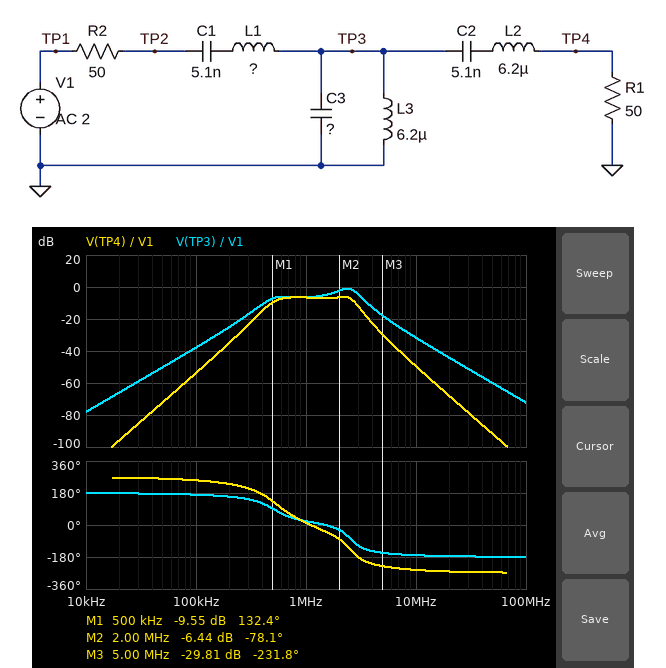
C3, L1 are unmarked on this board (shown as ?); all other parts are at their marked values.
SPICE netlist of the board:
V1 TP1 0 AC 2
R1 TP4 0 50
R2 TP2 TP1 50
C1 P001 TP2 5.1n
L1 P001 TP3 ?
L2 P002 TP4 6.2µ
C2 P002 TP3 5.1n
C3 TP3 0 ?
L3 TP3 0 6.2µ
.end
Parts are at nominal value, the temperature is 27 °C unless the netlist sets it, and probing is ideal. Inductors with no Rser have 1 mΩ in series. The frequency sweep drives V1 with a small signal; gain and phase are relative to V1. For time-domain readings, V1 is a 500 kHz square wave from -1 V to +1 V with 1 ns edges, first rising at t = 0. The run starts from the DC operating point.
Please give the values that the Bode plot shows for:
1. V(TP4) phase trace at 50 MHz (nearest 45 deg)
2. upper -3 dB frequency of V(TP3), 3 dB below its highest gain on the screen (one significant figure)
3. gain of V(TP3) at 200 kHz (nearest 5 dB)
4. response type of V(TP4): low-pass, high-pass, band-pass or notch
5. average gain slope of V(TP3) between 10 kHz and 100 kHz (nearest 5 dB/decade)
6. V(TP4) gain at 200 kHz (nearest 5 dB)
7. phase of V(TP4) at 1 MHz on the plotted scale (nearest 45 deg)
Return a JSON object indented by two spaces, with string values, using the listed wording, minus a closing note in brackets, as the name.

{
  "V(TP4) phase trace at 50 MHz": "-270 deg",
  "upper -3 dB frequency of V(TP3), 3 dB below its highest gain on the screen": "3 MHz",
  "gain of V(TP3) at 200 kHz": "-25 dB",
  "response type of V(TP4): low-pass, high-pass, band-pass or notch": "band-pass",
  "average gain slope of V(TP3) between 10 kHz and 100 kHz": "40 dB/decade",
  "V(TP4) gain at 200 kHz": "-35 dB",
  "phase of V(TP4) at 1 MHz on the plotted scale": "0 deg"
}
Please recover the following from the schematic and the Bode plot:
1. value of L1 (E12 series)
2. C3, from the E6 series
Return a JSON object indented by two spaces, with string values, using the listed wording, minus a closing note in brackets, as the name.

{
  "value of L1": "4.7 µH",
  "C3, from the E6 series": "2.2 nF"
}
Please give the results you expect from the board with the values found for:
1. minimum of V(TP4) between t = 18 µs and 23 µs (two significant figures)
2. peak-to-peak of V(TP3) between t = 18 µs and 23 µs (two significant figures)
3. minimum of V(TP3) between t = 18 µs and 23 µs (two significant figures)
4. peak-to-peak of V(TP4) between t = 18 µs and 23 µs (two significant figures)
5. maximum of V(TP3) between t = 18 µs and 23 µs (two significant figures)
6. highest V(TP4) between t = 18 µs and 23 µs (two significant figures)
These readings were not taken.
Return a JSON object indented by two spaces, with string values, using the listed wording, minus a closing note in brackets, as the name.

{
  "minimum of V(TP4) between t = 18 µs and 23 µs": "-510 mV",
  "peak-to-peak of V(TP3) between t = 18 µs and 23 µs": "2.0 V",
  "minimum of V(TP3) between t = 18 µs and 23 µs": "-1.0 V",
  "peak-to-peak of V(TP4) between t = 18 µs and 23 µs": "1.0 V",
  "maximum of V(TP3) between t = 18 µs and 23 µs": "1.0 V",
  "highest V(TP4) between t = 18 µs and 23 µs": "510 mV"
}
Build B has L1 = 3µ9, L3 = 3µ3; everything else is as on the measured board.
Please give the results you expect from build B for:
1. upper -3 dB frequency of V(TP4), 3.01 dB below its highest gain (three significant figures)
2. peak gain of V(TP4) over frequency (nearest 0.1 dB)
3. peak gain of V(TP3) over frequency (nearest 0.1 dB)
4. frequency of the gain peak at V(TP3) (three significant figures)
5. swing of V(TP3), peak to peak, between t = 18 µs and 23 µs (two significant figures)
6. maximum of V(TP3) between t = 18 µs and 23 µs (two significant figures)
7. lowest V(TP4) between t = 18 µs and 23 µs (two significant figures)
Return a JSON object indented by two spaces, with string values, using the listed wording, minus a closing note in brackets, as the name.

{
  "upper -3 dB frequency of V(TP4), 3.01 dB below its highest gain": "3.11 MHz",
  "peak gain of V(TP4) over frequency": "-6.6 dB",
  "peak gain of V(TP3) over frequency": "0 dB",
  "frequency of the gain peak at V(TP3)": "2.75 MHz",
  "swing of V(TP3), peak to peak, between t = 18 µs and 23 µs": "1.4 V",
  "maximum of V(TP3) between t = 18 µs and 23 µs": "690 mV",
  "lowest V(TP4) between t = 18 µs and 23 µs": "-360 mV"
}
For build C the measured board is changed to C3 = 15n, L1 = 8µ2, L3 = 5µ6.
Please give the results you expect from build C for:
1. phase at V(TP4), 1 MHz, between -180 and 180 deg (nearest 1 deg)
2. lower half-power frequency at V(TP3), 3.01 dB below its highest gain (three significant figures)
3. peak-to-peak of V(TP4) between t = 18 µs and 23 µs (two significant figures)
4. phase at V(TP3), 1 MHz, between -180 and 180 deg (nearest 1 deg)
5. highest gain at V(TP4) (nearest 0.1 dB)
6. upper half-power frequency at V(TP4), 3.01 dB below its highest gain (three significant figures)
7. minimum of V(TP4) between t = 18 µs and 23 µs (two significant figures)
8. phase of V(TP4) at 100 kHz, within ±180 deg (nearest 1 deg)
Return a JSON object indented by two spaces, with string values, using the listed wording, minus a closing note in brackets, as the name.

{
  "phase at V(TP4), 1 MHz, between -180 and 180 deg": "-88 deg",
  "lower half-power frequency at V(TP3), 3.01 dB below its highest gain": "381 kHz",
  "peak-to-peak of V(TP4) between t = 18 µs and 23 µs": "1.1 V",
  "phase at V(TP3), 1 MHz, between -180 and 180 deg": "-79 deg",
  "highest gain at V(TP4)": "-6.0 dB",
  "upper half-power frequency at V(TP4), 3.01 dB below its highest gain": "755 kHz",
  "minimum of V(TP4) between t = 18 µs and 23 µs": "-560 mV",
  "phase of V(TP4) at 100 kHz, within ±180 deg": "-109 deg"
}
